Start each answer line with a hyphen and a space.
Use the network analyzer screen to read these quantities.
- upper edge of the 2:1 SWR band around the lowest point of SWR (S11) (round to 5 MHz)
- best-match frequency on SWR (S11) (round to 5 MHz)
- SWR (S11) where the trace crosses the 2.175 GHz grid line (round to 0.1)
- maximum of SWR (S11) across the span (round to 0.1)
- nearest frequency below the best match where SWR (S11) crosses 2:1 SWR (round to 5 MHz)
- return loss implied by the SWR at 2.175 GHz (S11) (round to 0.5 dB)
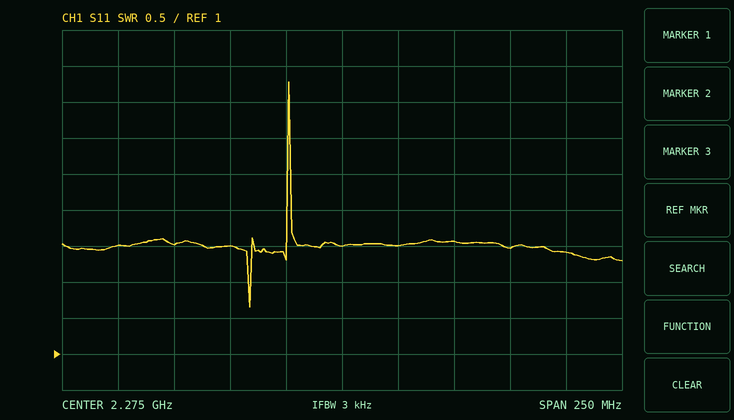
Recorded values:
- 2.235 GHz
- 2.235 GHz
- 2.5
- 4.8
- 2.235 GHz
- 7.5 dB
